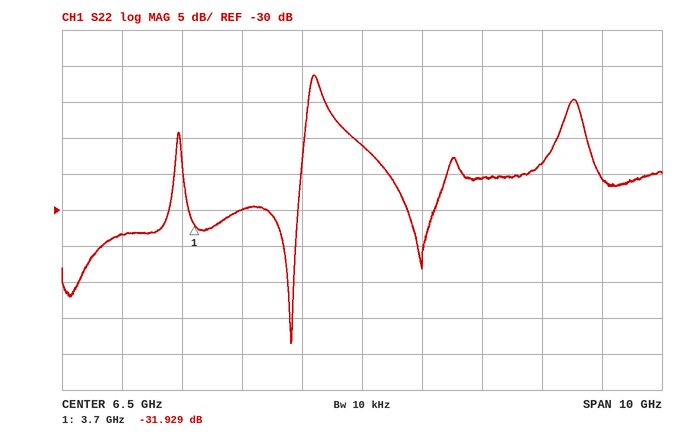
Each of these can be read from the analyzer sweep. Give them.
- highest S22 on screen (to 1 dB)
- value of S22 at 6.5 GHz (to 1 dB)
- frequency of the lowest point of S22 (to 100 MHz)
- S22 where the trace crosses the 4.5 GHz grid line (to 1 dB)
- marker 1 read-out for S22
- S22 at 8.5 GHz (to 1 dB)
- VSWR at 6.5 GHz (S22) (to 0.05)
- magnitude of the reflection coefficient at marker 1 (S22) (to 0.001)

-11 dB
-21 dB
5.3 GHz
-30 dB
-31.929 dB
-26 dB
1.20
0.025
